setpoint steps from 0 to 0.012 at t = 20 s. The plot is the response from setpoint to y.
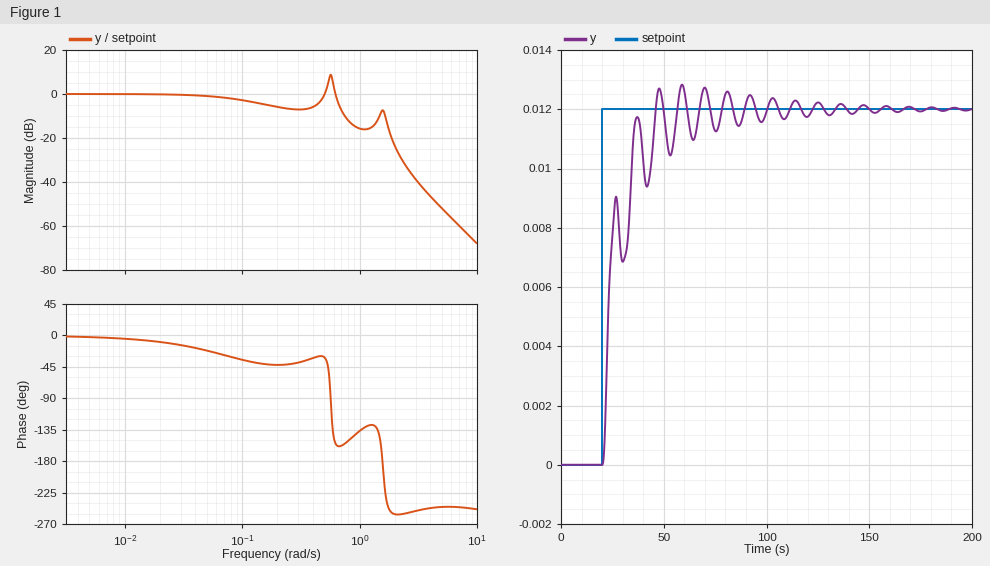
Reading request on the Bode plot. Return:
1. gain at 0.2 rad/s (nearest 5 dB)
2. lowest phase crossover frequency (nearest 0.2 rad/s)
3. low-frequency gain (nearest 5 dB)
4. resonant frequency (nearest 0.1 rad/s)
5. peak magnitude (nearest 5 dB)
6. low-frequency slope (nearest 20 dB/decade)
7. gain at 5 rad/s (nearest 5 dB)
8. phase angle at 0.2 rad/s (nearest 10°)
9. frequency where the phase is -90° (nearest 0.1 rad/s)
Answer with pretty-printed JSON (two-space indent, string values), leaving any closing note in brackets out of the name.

{
  "gain at 0.2 rad/s": "-5 dB",
  "lowest phase crossover frequency": "1.6 rad/s",
  "low-frequency gain": "0 dB",
  "resonant frequency": "0.6 rad/s",
  "peak magnitude": "10 dB",
  "low-frequency slope": "0 dB/decade",
  "gain at 5 rad/s": "-50 dB",
  "phase angle at 0.2 rad/s": "-40°",
  "frequency where the phase is -90°": "0.6 rad/s"
}
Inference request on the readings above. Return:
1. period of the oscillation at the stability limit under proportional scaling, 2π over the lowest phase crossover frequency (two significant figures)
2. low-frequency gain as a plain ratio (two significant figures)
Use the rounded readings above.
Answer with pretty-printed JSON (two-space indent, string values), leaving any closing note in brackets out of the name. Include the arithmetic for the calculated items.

{
  "period of the oscillation at the stability limit under proportional scaling, 2π over the lowest phase crossover frequency": "2π / 1.6 = 3.9 s",
  "low-frequency gain as a plain ratio": "10^(0 / 20) = 1.0"
}
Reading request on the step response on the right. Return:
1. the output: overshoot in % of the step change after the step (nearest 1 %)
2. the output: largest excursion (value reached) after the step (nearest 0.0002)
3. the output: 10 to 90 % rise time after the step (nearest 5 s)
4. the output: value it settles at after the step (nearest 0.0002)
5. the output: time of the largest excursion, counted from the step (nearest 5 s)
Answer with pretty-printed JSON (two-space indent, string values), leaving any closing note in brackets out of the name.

{
  "the output: overshoot in % of the step change after the step": "7 %",
  "the output: largest excursion (value reached) after the step": "0.0128",
  "the output: 10 to 90 % rise time after the step": "15 s",
  "the output: value it settles at after the step": "0.0120",
  "the output: time of the largest excursion, counted from the step": "40 s"
}
